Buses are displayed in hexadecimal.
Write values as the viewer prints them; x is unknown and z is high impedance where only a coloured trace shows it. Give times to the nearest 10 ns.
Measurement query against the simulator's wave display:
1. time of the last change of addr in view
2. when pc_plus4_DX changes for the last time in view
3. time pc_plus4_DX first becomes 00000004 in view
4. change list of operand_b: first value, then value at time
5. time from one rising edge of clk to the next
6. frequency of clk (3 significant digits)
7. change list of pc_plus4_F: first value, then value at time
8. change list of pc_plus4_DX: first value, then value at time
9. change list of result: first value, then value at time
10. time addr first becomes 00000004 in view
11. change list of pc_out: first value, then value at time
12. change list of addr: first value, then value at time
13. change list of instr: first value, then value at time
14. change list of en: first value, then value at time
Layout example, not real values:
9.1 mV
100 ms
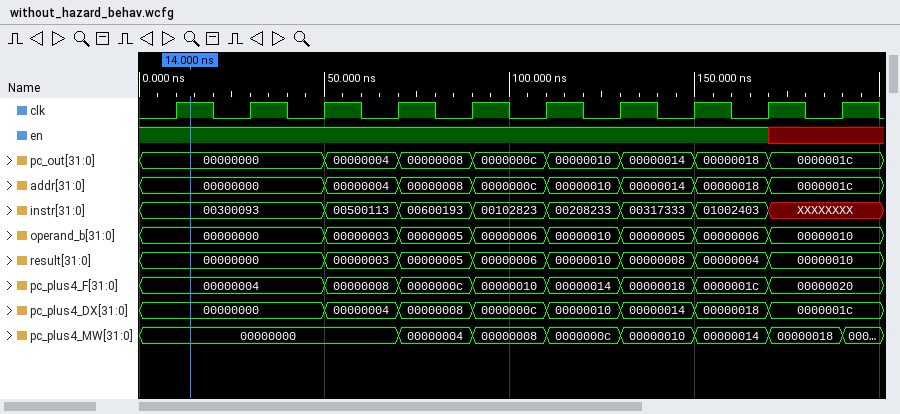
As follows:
170 ns
170 ns
50 ns
00000000, 00000003 at 50 ns, 00000005 at 70 ns, 00000006 at 90 ns, 00000010 at 110 ns, 00000005 at 130 ns, 00000006 at 150 ns, 00000010 at 170 ns
20 ns
50.0 MHz
00000004, 00000008 at 50 ns, 0000000c at 70 ns, 00000010 at 90 ns, 00000014 at 110 ns, 00000018 at 130 ns, 0000001c at 150 ns, 00000020 at 170 ns
00000000, 00000004 at 50 ns, 00000008 at 70 ns, 0000000c at 90 ns, 00000010 at 110 ns, 00000014 at 130 ns, 00000018 at 150 ns, 0000001c at 170 ns
00000000, 00000003 at 50 ns, 00000005 at 70 ns, 00000006 at 90 ns, 00000010 at 110 ns, 00000008 at 130 ns, 00000004 at 150 ns, 00000010 at 170 ns
50 ns
00000000, 00000004 at 50 ns, 00000008 at 70 ns, 0000000c at 90 ns, 00000010 at 110 ns, 00000014 at 130 ns, 00000018 at 150 ns, 0000001c at 170 ns
00000000, 00000004 at 50 ns, 00000008 at 70 ns, 0000000c at 90 ns, 00000010 at 110 ns, 00000014 at 130 ns, 00000018 at 150 ns, 0000001c at 170 ns
00300093, 00500113 at 50 ns, 00600193 at 70 ns, 00102823 at 90 ns, 00208233 at 110 ns, 00317333 at 130 ns, 01002403 at 150 ns, XXXXXXXX at 170 ns
1, x at 170 ns
